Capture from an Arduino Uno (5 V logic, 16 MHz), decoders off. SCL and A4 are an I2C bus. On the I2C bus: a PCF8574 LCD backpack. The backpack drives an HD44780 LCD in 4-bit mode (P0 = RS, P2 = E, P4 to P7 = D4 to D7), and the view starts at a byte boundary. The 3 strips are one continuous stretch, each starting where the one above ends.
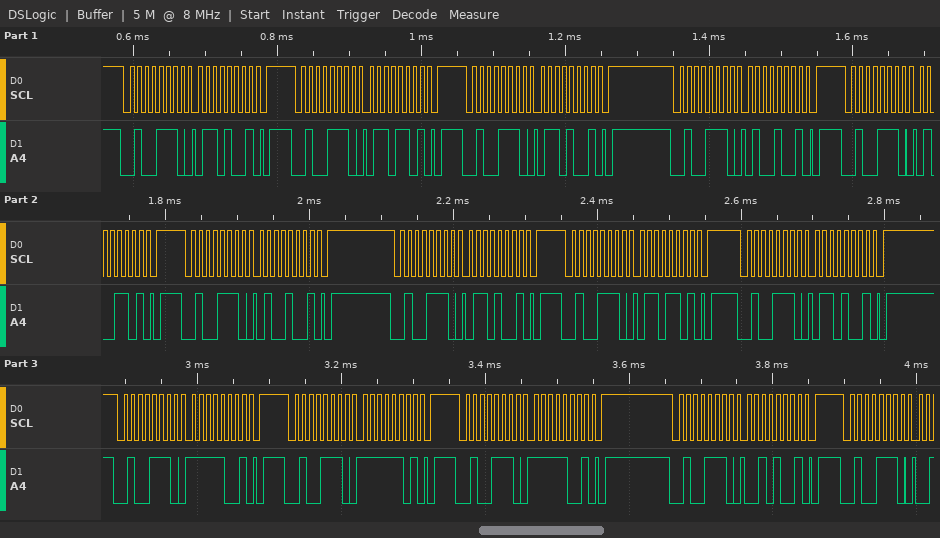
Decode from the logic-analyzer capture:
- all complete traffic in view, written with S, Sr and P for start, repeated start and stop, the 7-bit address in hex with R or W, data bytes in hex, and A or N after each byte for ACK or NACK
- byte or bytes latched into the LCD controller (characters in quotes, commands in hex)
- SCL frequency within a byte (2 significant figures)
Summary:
S 27W A 69 A P S 27W A 6D A P S 27W A 69 A P S 27W A 49 A P S 27W A 4D A P S 27W A 49 A P S 27W A 69 A P S 27W A 6D A P S 27W A 69 A P S 27W A F9 A P S 27W A FD A P S 27W A F9 A P S 27W A 29 A P S 27W A
'd' 'o'
100 kHz
